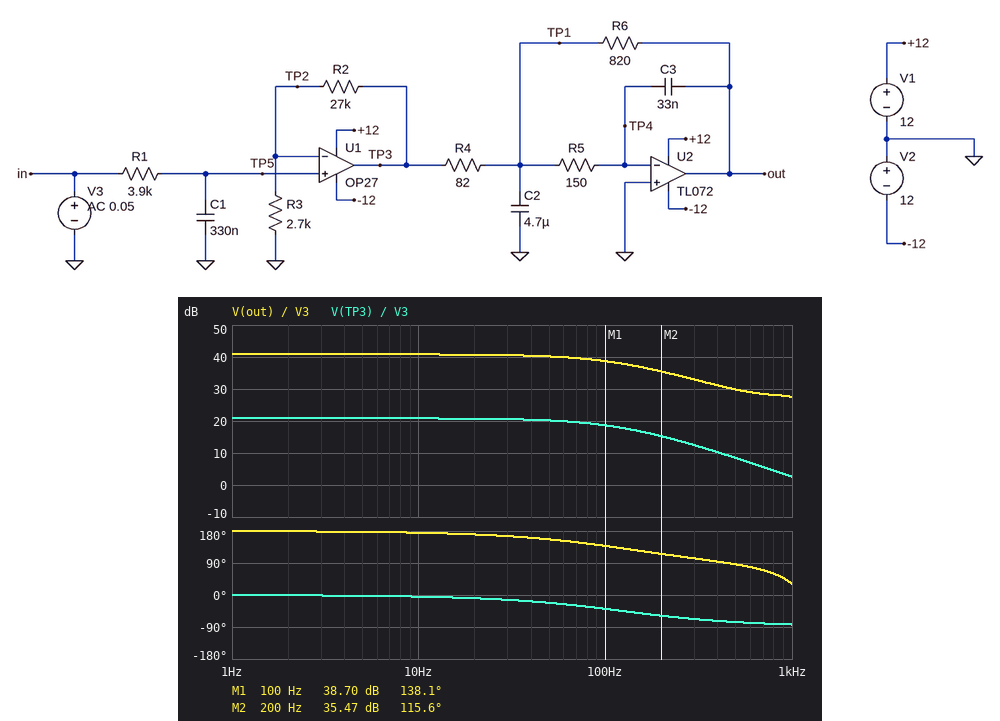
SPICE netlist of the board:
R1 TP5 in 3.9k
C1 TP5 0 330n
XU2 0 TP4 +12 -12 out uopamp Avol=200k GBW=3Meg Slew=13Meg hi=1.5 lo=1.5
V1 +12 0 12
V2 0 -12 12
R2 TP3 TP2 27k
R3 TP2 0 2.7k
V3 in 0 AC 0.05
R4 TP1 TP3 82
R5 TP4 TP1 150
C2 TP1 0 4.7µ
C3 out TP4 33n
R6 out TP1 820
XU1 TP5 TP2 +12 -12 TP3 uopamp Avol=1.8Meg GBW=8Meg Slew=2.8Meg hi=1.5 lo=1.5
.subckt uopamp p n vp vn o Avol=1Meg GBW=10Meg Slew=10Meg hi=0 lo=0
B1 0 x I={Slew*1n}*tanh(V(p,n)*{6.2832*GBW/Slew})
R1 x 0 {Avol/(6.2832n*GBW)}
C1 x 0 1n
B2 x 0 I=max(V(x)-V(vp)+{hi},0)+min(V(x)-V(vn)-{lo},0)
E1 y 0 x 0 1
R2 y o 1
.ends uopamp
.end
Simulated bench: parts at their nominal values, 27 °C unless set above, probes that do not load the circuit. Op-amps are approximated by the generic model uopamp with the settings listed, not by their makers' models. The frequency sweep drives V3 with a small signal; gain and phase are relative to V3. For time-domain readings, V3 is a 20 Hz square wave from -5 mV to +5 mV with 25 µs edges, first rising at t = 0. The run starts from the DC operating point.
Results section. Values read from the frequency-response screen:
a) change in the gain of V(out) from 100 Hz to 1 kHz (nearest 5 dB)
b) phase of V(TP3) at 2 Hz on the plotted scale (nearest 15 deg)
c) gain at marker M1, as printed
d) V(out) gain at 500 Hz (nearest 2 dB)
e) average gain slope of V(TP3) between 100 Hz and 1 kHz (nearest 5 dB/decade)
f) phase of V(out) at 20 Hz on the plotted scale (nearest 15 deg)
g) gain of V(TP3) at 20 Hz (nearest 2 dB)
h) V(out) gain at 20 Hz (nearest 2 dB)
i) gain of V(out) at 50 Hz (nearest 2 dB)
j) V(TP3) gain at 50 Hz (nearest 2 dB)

-10 dB
0 deg
38.70 dB
30 dB
-15 dB/decade
165 deg
20 dB
40 dB
40 dB
20 dB
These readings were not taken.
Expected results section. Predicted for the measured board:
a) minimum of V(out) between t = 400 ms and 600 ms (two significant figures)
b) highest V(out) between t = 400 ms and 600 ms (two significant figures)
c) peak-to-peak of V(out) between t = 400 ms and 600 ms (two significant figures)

-550 mV
550 mV
1.1 V
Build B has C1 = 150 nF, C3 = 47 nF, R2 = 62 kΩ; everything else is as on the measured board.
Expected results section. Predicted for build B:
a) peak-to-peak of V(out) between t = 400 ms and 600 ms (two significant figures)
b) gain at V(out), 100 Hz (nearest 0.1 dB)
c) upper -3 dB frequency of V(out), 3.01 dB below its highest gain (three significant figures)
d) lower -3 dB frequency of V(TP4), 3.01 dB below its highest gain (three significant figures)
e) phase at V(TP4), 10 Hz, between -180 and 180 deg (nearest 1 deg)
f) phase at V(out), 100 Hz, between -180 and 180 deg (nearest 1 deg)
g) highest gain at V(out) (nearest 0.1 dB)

2.4 V
47.1 dB
317 Hz
458 Hz
31 deg
156 deg
47.6 dB
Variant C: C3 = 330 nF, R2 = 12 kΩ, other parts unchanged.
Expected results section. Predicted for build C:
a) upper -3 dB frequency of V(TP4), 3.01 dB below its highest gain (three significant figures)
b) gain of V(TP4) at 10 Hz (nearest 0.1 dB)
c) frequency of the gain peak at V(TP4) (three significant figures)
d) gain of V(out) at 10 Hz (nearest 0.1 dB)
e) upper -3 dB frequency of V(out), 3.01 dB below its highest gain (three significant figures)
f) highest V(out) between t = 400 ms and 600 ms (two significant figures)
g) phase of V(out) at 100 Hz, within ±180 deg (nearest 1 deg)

378 Hz
-69.7 dB
176 Hz
34.7 dB
108 Hz
270 mV
112 deg
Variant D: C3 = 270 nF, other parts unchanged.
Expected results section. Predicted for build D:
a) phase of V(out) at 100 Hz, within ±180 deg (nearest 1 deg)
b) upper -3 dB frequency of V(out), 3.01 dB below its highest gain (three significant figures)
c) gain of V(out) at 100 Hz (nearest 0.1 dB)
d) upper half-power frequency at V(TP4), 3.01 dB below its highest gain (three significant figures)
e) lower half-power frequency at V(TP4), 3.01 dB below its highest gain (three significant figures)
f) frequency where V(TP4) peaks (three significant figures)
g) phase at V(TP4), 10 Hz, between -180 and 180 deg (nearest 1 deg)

117 deg
115 Hz
38.4 dB
427 Hz
78.1 Hz
202 Hz
27 deg
